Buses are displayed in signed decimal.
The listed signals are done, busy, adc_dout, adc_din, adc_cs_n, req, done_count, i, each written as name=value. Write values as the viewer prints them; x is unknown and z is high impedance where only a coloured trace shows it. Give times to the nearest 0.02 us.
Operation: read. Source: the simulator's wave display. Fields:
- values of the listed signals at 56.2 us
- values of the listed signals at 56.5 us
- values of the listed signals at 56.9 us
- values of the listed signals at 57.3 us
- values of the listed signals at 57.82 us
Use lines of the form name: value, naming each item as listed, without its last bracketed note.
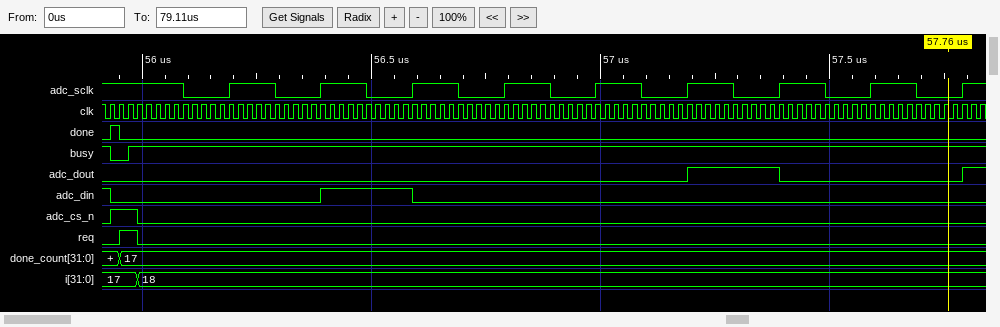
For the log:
values of the listed signals at 56.2 us: done=0, busy=1, adc_dout=0, adc_din=0, adc_cs_n=0, req=0, done_count=17, i=18
values of the listed signals at 56.5 us: done=0, busy=1, adc_dout=0, adc_din=1, adc_cs_n=0, req=0, done_count=17, i=18
values of the listed signals at 56.9 us: done=0, busy=1, adc_dout=0, adc_din=0, adc_cs_n=0, req=0, done_count=17, i=18
values of the listed signals at 57.3 us: done=0, busy=1, adc_dout=1, adc_din=0, adc_cs_n=0, req=0, done_count=17, i=18
values of the listed signals at 57.82 us: done=0, busy=1, adc_dout=1, adc_din=0, adc_cs_n=0, req=0, done_count=17, i=18
